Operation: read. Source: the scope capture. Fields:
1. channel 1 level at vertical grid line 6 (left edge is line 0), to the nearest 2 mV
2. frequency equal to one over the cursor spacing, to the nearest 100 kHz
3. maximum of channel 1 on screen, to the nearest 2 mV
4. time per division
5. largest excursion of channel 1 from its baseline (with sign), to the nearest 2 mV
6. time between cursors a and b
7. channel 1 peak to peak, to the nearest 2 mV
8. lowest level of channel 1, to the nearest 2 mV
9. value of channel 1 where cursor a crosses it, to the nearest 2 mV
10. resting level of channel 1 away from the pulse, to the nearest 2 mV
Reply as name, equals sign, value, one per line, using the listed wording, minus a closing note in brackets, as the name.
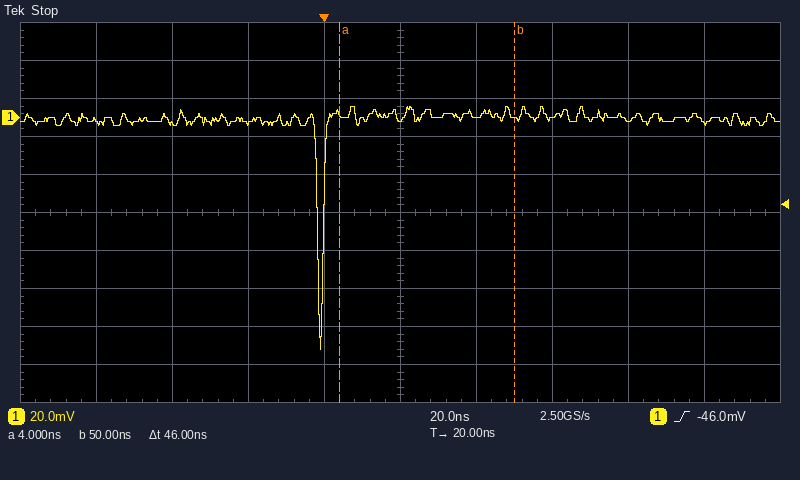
channel 1 level at vertical grid line 6 (left edge is line 0), to the nearest 2 mV = 0 mV
frequency equal to one over the cursor spacing, to the nearest 100 kHz = 21.7 MHz
maximum of channel 1 on screen, to the nearest 2 mV = 6 mV
time per division = 20 ns
largest excursion of channel 1 from its baseline (with sign), to the nearest 2 mV = -122 mV
time between cursors a and b = 46 ns
channel 1 peak to peak, to the nearest 2 mV = 128 mV
lowest level of channel 1, to the nearest 2 mV = -122 mV
value of channel 1 where cursor a crosses it, to the nearest 2 mV = 2 mV
resting level of channel 1 away from the pulse, to the nearest 2 mV = 0 mV
